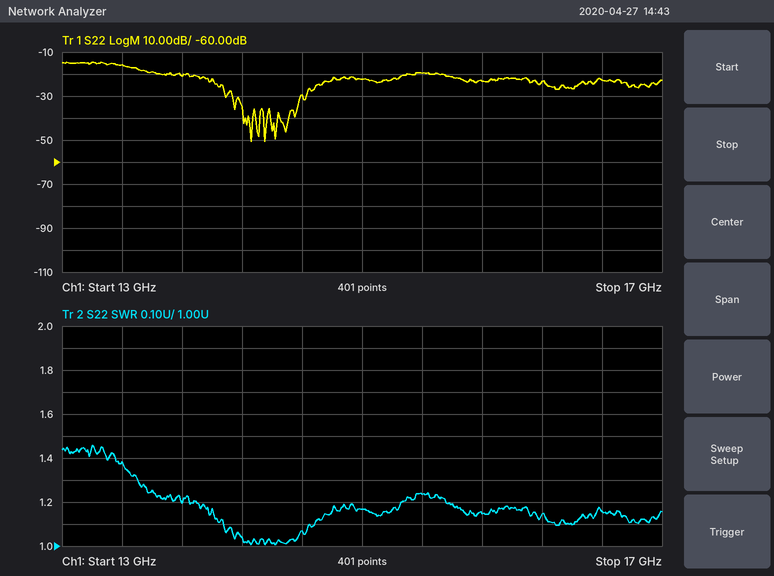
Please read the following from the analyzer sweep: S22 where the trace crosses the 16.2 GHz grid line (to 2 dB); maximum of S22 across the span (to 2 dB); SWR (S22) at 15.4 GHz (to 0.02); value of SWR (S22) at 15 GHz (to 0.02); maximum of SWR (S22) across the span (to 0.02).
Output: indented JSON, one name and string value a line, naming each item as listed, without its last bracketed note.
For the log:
{
  "S22 where the trace crosses the 16.2 GHz grid line": "-24 dB",
  "maximum of S22 across the span": "-14 dB",
  "SWR (S22) at 15.4 GHz": "1.24",
  "value of SWR (S22) at 15 GHz": "1.16",
  "maximum of SWR (S22) across the span": "1.46"
}
